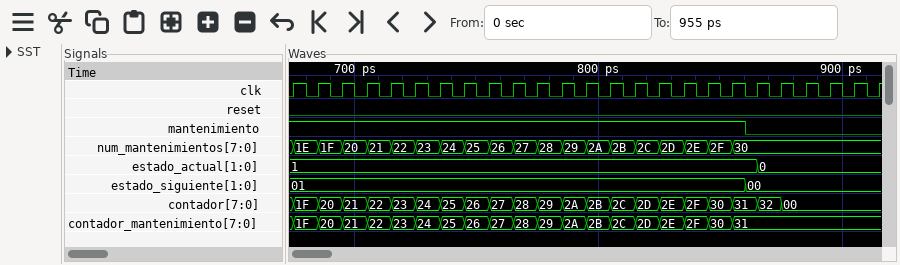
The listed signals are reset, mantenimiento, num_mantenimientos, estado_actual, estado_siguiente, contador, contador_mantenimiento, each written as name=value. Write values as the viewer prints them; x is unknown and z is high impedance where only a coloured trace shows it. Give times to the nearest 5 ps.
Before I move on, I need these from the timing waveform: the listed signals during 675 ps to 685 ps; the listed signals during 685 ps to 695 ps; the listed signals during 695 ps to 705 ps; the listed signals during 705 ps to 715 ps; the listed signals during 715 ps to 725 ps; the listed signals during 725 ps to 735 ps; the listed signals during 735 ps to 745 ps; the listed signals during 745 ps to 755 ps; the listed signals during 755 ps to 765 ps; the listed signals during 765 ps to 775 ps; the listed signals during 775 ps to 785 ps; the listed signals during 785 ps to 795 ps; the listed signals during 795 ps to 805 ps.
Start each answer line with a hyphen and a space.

- reset=0, mantenimiento=1, num_mantenimientos=1E, estado_actual=1, estado_siguiente=01, contador=1F, contador_mantenimiento=1F
- reset=0, mantenimiento=1, num_mantenimientos=1F, estado_actual=1, estado_siguiente=01, contador=20, contador_mantenimiento=20
- reset=0, mantenimiento=1, num_mantenimientos=20, estado_actual=1, estado_siguiente=01, contador=21, contador_mantenimiento=21
- reset=0, mantenimiento=1, num_mantenimientos=21, estado_actual=1, estado_siguiente=01, contador=22, contador_mantenimiento=22
- reset=0, mantenimiento=1, num_mantenimientos=22, estado_actual=1, estado_siguiente=01, contador=23, contador_mantenimiento=23
- reset=0, mantenimiento=1, num_mantenimientos=23, estado_actual=1, estado_siguiente=01, contador=24, contador_mantenimiento=24
- reset=0, mantenimiento=1, num_mantenimientos=24, estado_actual=1, estado_siguiente=01, contador=25, contador_mantenimiento=25
- reset=0, mantenimiento=1, num_mantenimientos=25, estado_actual=1, estado_siguiente=01, contador=26, contador_mantenimiento=26
- reset=0, mantenimiento=1, num_mantenimientos=26, estado_actual=1, estado_siguiente=01, contador=27, contador_mantenimiento=27
- reset=0, mantenimiento=1, num_mantenimientos=27, estado_actual=1, estado_siguiente=01, contador=28, contador_mantenimiento=28
- reset=0, mantenimiento=1, num_mantenimientos=28, estado_actual=1, estado_siguiente=01, contador=29, contador_mantenimiento=29
- reset=0, mantenimiento=1, num_mantenimientos=29, estado_actual=1, estado_siguiente=01, contador=2A, contador_mantenimiento=2A
- reset=0, mantenimiento=1, num_mantenimientos=2A, estado_actual=1, estado_siguiente=01, contador=2B, contador_mantenimiento=2B
